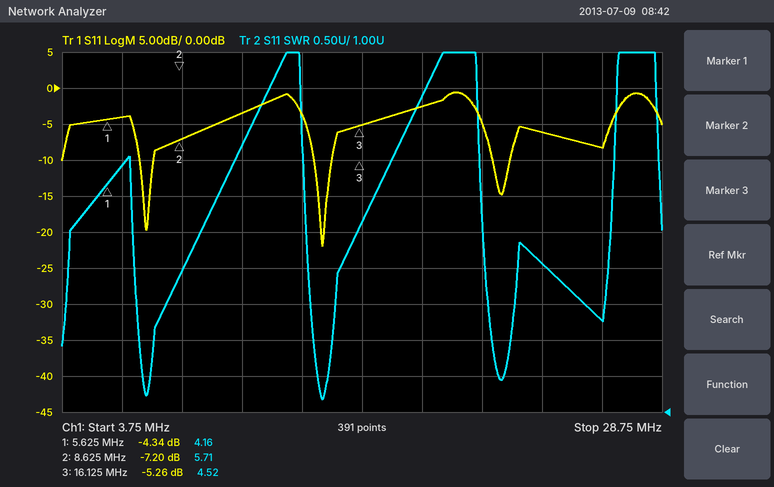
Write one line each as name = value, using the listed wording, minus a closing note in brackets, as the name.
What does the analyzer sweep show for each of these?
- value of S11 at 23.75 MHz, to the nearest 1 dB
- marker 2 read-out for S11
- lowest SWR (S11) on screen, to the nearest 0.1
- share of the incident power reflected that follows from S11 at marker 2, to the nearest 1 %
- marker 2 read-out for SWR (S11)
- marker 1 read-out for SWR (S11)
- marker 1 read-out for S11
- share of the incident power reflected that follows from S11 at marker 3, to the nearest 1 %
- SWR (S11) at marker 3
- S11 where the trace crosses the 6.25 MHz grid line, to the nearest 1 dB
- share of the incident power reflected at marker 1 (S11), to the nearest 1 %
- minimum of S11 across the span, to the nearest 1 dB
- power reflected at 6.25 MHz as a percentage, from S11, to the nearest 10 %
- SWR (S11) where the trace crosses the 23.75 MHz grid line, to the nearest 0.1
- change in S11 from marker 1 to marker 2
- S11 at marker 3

value of S11 at 23.75 MHz, to the nearest 1 dB = -6 dB
marker 2 read-out for S11 = -7.20 dB
lowest SWR (S11) on screen, to the nearest 0.1 = 1.2
share of the incident power reflected that follows from S11 at marker 2, to the nearest 1 % = 19 %
marker 2 read-out for SWR = 5.71
marker 1 read-out for SWR = 4.16
marker 1 read-out for S11 = -4.34 dB
share of the incident power reflected that follows from S11 at marker 3, to the nearest 1 % = 30 %
SWR (S11) at marker 3 = 4.52
S11 where the trace crosses the 6.25 MHz grid line, to the nearest 1 dB = -4 dB
share of the incident power reflected at marker 1 (S11), to the nearest 1 % = 37 %
minimum of S11 across the span, to the nearest 1 dB = -22 dB
power reflected at 6.25 MHz as a percentage, from S11, to the nearest 10 % = 40 %
SWR (S11) where the trace crosses the 23.75 MHz grid line, to the nearest 0.1 = 3.1
change in S11 from marker 1 to marker 2 = -2.86 dB
S11 at marker 3 = -5.26 dB
